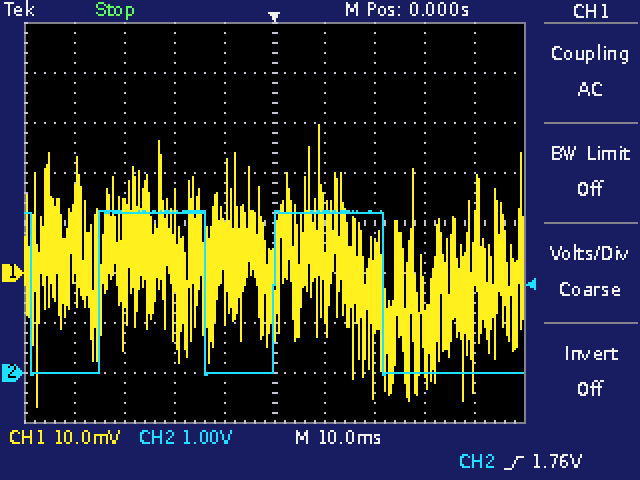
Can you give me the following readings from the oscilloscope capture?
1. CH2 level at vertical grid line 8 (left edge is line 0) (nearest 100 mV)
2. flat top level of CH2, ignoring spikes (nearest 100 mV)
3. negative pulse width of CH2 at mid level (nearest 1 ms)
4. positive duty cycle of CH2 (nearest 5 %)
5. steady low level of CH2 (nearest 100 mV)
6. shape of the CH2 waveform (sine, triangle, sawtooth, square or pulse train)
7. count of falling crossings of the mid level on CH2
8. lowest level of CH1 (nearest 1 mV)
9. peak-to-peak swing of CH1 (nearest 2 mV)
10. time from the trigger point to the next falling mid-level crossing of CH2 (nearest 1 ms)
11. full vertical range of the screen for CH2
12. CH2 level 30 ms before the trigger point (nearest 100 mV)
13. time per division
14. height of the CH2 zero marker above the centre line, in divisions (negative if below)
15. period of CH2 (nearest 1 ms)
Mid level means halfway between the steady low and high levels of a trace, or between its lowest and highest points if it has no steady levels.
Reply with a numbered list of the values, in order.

1. 0.0 V
2. 3.2 V
3. 14 ms
4. 60 %
5. 0.0 V
6. pulse train
7. 3
8. -27 mV
9. 56 mV
10. 22 ms
11. 8 V
12. 3.2 V
13. 10 ms
14. -3.0 div
15. 35 ms
